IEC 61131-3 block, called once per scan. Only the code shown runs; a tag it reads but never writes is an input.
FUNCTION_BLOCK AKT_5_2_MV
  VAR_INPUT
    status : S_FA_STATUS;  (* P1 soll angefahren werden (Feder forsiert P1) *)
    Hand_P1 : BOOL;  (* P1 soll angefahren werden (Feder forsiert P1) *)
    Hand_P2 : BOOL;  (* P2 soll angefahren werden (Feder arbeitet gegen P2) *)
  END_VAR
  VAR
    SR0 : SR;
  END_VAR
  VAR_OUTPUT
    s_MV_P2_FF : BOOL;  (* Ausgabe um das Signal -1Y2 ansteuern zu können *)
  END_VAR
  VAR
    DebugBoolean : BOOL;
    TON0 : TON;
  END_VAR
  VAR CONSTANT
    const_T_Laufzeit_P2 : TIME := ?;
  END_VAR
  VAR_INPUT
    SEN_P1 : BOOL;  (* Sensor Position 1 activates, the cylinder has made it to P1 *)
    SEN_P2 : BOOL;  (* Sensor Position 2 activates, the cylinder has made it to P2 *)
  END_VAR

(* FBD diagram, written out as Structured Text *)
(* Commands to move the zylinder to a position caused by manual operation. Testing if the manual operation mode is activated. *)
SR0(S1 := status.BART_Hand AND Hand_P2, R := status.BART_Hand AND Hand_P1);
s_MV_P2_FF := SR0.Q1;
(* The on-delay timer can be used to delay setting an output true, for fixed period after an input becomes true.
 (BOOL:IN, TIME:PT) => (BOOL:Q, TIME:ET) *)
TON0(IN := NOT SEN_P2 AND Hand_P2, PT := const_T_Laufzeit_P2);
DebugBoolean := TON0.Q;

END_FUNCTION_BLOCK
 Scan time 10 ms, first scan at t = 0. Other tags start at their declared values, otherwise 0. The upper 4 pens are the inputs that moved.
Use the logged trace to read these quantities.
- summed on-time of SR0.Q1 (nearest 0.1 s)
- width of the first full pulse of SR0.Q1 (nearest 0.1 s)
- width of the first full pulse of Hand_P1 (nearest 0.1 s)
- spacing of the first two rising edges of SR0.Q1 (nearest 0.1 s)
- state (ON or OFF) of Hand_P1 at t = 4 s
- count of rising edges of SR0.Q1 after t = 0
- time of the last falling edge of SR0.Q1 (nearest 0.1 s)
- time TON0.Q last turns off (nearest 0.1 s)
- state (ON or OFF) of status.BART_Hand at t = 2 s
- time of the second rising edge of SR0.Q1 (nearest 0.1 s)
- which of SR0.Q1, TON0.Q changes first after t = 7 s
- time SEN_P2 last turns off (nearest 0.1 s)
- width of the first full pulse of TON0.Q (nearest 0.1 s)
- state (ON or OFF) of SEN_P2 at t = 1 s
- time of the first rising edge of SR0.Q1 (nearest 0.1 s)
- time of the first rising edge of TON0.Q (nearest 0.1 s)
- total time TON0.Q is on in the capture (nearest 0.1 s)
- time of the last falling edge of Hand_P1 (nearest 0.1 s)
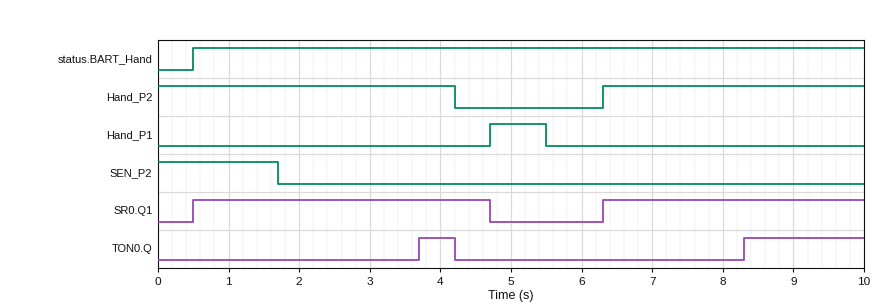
7.9 s
4.2 s
0.8 s
5.8 s
OFF
2
4.7 s
4.2 s
ON
6.3 s
TON0.Q
1.7 s
0.5 s
ON
0.5 s
3.7 s
2.2 s
5.5 s
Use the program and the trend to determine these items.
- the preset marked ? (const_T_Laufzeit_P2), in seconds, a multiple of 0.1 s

2.0 s
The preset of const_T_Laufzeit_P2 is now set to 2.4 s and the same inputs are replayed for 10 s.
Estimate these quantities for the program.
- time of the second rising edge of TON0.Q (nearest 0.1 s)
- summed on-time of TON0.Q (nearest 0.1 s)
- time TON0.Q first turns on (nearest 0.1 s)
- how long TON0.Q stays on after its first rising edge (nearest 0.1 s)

8.7 s
1.4 s
4.1 s
0.1 s
